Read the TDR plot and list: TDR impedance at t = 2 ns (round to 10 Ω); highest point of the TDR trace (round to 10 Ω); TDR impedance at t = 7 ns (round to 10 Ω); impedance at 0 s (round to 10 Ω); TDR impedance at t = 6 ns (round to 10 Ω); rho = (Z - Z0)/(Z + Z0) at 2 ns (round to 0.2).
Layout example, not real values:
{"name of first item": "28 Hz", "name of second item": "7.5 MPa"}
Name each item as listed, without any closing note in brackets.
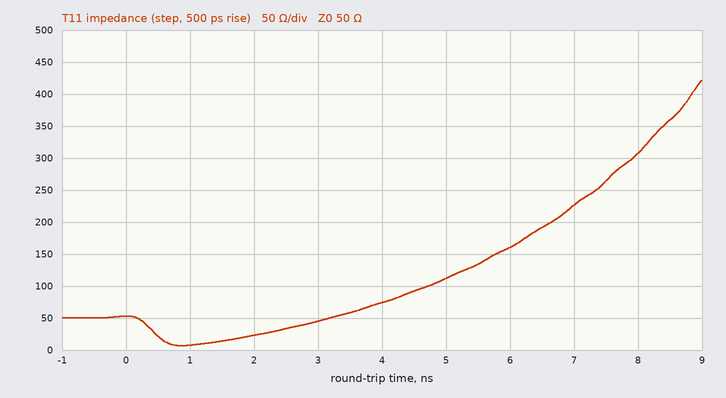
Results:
{"TDR impedance at t = 2 ns": "20 Ω", "highest point of the TDR trace": "420 Ω", "TDR impedance at t = 7 ns": "230 Ω", "impedance at 0 s": "50 Ω", "TDR impedance at t = 6 ns": "160 Ω", "rho = (Z - Z0)/(Z + Z0) at 2 ns": "-0.4"}
